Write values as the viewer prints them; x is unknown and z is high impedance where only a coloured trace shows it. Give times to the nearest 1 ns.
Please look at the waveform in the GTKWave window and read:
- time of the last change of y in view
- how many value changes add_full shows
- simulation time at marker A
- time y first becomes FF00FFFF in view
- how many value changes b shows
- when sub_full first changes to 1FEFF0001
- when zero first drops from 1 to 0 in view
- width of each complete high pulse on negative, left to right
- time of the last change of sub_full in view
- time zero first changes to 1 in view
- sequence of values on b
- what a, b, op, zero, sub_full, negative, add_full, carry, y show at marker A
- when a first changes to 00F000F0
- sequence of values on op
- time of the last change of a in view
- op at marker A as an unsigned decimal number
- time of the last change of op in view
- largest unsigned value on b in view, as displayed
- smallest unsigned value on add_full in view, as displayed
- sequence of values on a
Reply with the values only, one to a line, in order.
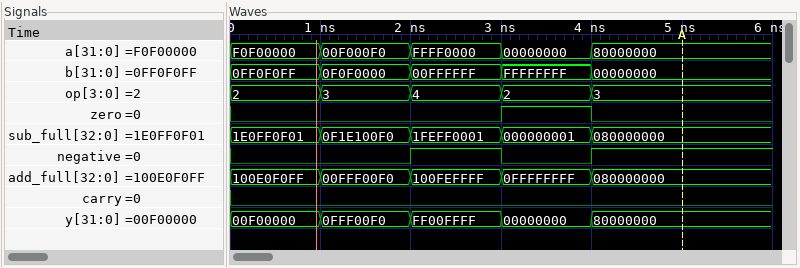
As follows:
4 ns
4
5 ns
2 ns
4
2 ns
4 ns
1 ns
4 ns
3 ns
0FF0F0FF, 0F0F0000, 00FFFFFF, FFFFFFFF, 00000000
a=80000000, b=00000000, op=3, zero=0, sub_full=080000000, negative=1, add_full=080000000, carry=0, y=80000000
1 ns
2, 3, 4, 2, 3
4 ns
3
4 ns
FFFFFFFF
00FFF00F0
F0F00000, 00F000F0, FFFF0000, 00000000, 80000000
